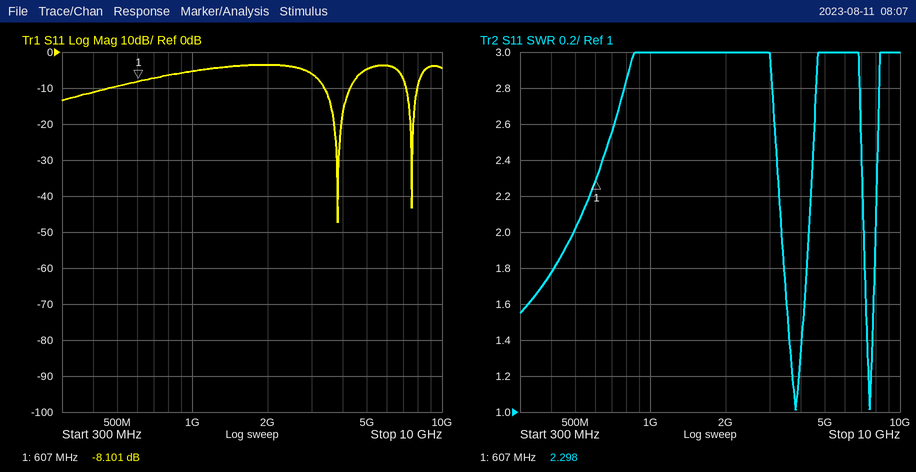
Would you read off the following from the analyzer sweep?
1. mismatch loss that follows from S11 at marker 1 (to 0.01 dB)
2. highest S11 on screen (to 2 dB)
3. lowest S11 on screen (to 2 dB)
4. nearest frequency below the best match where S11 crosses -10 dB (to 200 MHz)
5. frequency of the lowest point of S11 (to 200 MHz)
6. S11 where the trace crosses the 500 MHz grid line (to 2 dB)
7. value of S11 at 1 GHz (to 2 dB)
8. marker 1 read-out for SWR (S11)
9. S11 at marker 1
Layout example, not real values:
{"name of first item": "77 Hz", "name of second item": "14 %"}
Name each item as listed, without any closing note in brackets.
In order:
{"mismatch loss that follows from S11 at marker 1": "0.73 dB", "highest S11 on screen": "-4 dB", "lowest S11 on screen": "-48 dB", "nearest frequency below the best match where S11 crosses -10 dB": "3.4 GHz", "frequency of the lowest point of S11": "3.8 GHz", "S11 where the trace crosses the 500 MHz grid line": "-10 dB", "value of S11 at 1 GHz": "-6 dB", "marker 1 read-out for SWR": "2.298", "S11 at marker 1": "-8.101 dB"}
